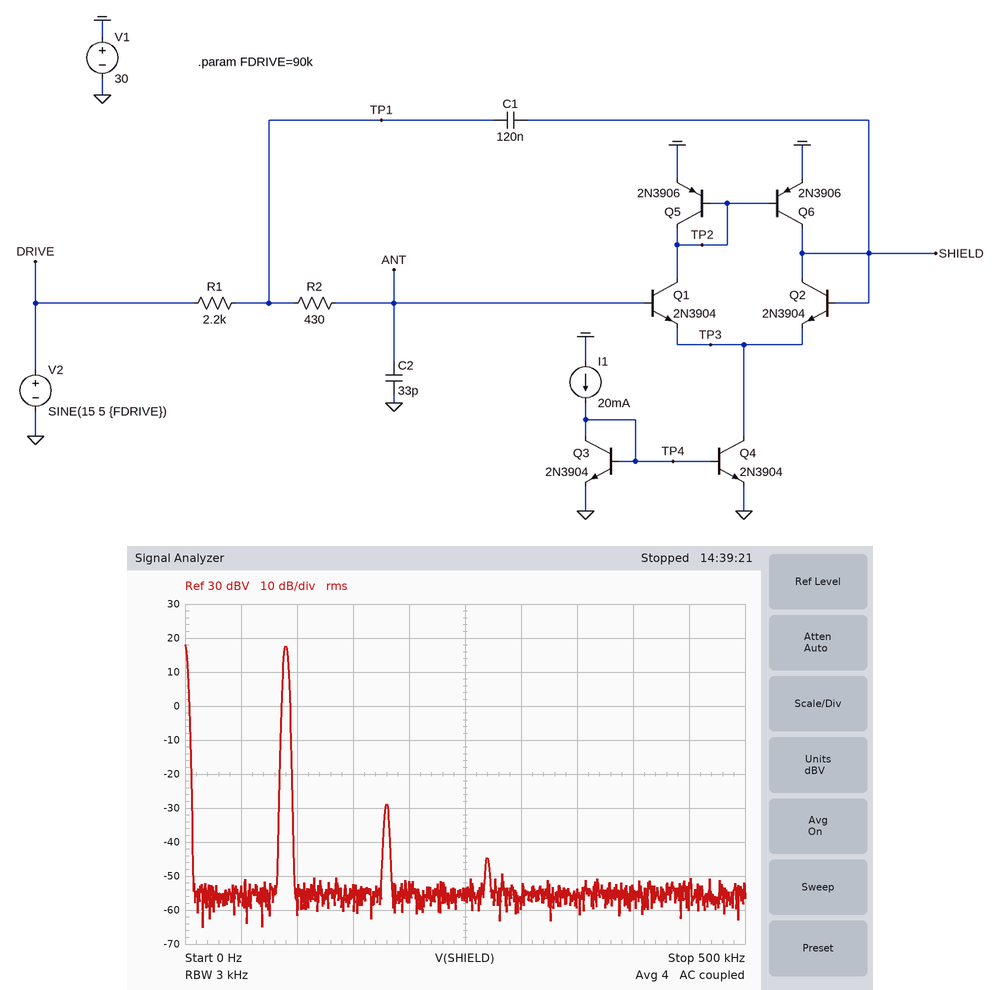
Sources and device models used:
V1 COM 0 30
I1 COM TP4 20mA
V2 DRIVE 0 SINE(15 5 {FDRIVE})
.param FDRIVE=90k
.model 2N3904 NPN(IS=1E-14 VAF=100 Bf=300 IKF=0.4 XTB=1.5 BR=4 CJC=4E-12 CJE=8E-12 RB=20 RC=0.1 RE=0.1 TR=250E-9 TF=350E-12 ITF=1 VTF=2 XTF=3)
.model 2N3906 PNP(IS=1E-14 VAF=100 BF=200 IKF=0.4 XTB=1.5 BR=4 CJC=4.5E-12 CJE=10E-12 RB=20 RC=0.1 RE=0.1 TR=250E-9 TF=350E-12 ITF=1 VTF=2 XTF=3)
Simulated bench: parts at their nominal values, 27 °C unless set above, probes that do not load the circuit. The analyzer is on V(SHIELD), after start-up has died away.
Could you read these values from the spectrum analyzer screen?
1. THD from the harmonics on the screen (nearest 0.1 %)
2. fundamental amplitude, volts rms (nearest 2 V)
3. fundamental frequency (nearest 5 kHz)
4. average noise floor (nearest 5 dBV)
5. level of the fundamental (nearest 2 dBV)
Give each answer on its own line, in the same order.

0.5 %
8 V
90 kHz
-55 dBV
18 dBV
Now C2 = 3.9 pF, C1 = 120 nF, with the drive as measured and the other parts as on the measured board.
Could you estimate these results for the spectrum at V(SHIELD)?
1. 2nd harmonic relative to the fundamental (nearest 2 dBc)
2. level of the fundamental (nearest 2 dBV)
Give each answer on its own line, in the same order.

-36 dBc
12 dBV
